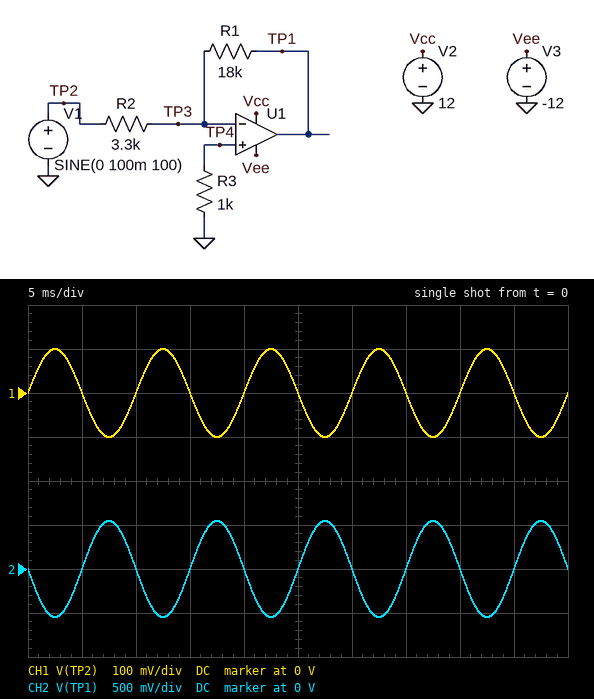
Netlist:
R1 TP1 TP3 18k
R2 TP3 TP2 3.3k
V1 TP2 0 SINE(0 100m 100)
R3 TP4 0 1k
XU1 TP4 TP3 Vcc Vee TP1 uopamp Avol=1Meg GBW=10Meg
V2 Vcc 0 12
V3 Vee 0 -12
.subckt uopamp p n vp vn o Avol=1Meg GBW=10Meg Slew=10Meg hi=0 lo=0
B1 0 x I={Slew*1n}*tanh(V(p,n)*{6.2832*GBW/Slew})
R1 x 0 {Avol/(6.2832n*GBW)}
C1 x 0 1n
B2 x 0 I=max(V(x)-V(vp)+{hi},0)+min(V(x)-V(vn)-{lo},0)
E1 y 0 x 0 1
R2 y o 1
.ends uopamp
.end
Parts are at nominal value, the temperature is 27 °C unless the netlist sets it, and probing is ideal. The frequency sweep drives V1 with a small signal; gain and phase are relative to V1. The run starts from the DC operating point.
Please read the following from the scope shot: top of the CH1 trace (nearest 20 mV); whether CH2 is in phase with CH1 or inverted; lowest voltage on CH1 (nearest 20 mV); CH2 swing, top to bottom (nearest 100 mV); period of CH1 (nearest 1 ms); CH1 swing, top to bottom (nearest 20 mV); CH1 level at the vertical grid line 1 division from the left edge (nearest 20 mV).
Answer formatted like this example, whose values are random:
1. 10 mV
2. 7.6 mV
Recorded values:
1. 100 mV
2. inverted
3. -100 mV
4. 1.1 V
5. 10 ms
6. 200 mV
7. 0 V
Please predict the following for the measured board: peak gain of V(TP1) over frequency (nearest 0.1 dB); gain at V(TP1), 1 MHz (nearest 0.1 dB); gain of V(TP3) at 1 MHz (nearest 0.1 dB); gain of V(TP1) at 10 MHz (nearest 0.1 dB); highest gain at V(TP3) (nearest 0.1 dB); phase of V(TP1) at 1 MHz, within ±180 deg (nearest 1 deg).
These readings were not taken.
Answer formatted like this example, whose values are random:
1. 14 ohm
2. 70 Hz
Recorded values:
1. 14.7 dB
2. 13.2 dB
3. -6.8 dB
4. -1.6 dB
5. -1.5 dB
6. 147 deg
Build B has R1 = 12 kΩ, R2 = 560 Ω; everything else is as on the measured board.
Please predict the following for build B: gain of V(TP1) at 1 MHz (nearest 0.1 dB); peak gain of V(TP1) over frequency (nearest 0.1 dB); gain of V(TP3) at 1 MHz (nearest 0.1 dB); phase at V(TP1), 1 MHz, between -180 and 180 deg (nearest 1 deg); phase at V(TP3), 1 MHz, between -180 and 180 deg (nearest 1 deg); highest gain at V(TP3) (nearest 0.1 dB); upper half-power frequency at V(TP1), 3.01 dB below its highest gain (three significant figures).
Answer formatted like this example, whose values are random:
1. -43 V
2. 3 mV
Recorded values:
1. 18.8 dB
2. 26.6 dB
3. -1.2 dB
4. 114 deg
5. 24 deg
6. -0.4 dB
7. 446 kHz
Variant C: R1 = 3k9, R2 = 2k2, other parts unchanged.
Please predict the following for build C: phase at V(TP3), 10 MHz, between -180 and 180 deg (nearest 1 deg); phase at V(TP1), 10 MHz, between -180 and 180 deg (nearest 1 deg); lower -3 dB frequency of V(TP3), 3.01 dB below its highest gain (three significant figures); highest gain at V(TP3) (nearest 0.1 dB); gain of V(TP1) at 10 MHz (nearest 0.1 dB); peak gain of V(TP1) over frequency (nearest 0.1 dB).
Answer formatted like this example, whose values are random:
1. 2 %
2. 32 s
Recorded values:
1. 20 deg
2. 110 deg
3. 3.61 MHz
4. -3.9 dB
5. -4.4 dB
6. 5.0 dB
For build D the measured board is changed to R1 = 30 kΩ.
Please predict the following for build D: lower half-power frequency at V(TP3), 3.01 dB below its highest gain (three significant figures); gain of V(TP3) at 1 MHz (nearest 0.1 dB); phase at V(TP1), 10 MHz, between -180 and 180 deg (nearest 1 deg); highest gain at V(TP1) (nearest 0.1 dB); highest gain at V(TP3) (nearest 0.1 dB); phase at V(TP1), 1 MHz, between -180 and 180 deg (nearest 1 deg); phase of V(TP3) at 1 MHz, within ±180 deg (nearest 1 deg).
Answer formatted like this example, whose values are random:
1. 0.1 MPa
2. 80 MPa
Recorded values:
1. 991 kHz
2. -3.9 dB
3. 96 deg
4. 19.2 dB
5. -0.9 dB
6. 135 deg
7. 45 deg
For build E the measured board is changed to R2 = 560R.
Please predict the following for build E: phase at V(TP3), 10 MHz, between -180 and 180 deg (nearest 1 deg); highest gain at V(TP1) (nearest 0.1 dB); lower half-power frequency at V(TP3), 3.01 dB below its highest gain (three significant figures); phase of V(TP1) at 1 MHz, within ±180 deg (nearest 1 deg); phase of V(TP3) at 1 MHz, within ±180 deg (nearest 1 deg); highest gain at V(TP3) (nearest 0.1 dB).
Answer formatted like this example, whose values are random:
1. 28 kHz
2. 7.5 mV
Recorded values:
1. 2 deg
2. 30.1 dB
3. 302 kHz
4. 107 deg
5. 17 deg
6. -0.3 dB
